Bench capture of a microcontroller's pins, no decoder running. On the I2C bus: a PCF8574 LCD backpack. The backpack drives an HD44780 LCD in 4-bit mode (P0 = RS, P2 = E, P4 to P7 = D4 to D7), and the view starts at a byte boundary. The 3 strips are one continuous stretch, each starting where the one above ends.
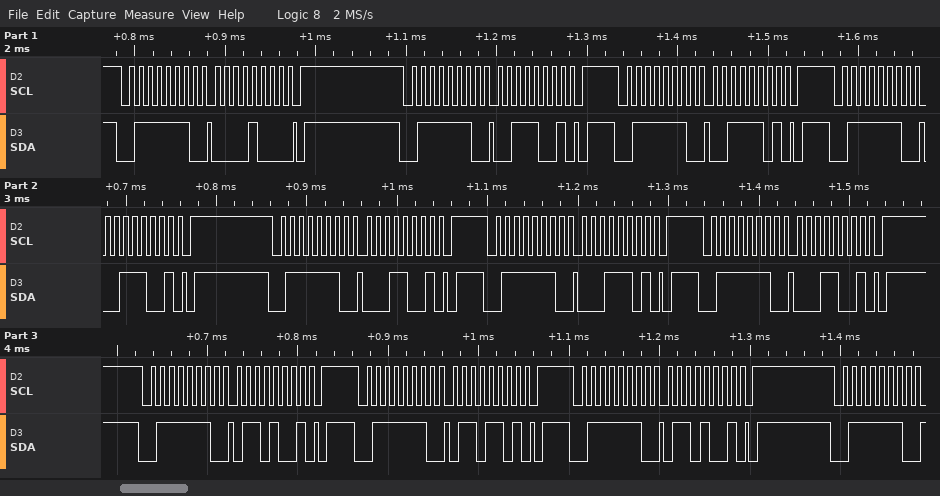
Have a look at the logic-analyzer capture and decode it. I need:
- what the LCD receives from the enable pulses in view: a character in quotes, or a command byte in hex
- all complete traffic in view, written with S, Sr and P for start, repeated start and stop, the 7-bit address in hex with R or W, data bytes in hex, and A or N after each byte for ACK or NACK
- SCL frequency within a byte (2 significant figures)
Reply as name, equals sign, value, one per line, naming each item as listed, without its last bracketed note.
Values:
what the LCD receives from the enable pulses in view: a character in quotes, or a command byte in hex = '1'
all complete traffic in view, written with S, Sr and P for start, repeated start and stop, the 7-bit address in hex with R or W, data bytes in hex, and A or N after each byte for ACK or NACK = S 3FW A 08 A P S 3FW A 39 A P S 3FW A 3D A P S 3FW A 39 A P S 3FW A 19 A P S 3FW A 1D A P S 3FW A 19 A P S 3FW A 69 A P S 3FW A 6D A P S 3FW A 69 A P S 3FW A
SCL frequency within a byte = 100 kHz
